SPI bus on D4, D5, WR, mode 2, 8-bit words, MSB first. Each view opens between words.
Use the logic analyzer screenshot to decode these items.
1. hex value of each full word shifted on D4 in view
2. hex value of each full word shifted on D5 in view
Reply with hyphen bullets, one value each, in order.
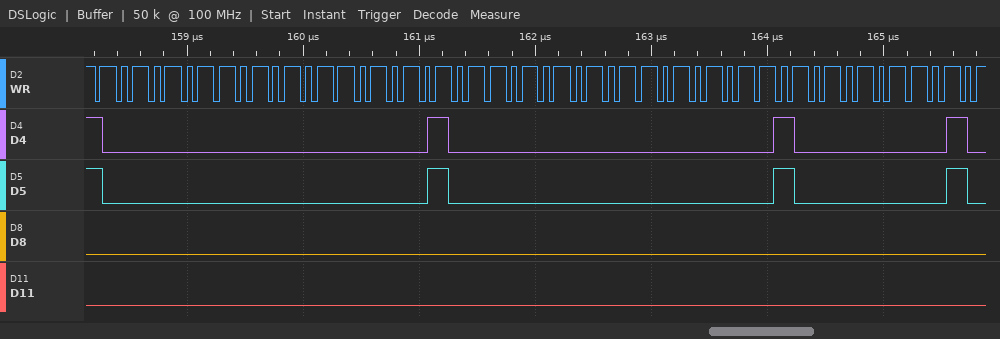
- 80, 00, 08, 00, 00, C0
- 80, 00, 08, 00, 00, C0
